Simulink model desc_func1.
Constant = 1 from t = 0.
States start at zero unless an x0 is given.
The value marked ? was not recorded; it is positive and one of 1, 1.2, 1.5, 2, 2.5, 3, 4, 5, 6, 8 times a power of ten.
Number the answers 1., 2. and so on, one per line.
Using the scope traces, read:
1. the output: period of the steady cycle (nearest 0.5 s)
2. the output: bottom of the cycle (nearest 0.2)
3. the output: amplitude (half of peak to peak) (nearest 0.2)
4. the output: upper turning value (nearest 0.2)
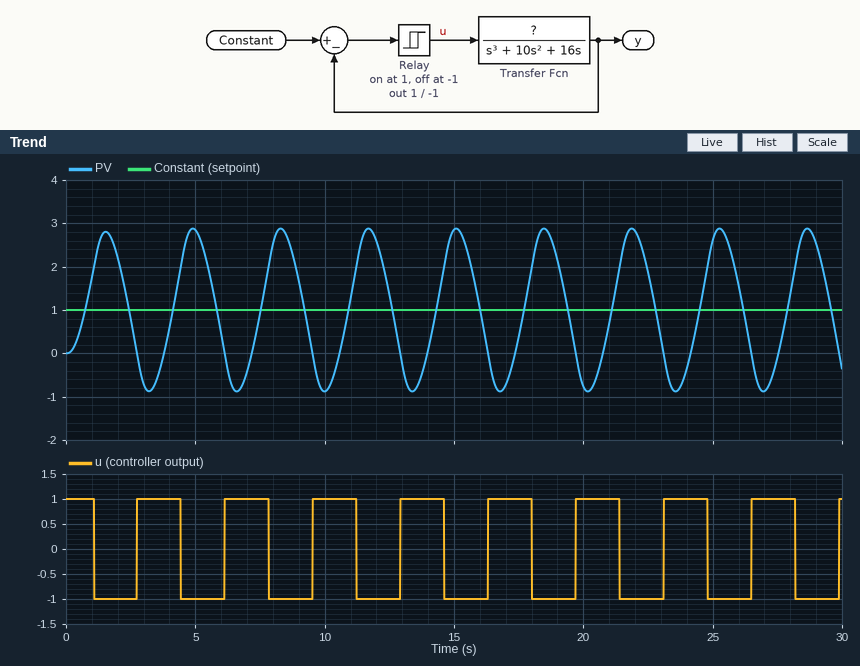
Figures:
1. 3.5 s
2. -0.8
3. 1.8
4. 2.8
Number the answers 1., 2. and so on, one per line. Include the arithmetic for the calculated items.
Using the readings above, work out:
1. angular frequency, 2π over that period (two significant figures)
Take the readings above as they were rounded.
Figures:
1. 2π / 3.5 = 1.8 rad/s
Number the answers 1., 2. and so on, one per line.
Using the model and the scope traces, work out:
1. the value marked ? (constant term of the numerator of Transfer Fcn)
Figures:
1. 60
